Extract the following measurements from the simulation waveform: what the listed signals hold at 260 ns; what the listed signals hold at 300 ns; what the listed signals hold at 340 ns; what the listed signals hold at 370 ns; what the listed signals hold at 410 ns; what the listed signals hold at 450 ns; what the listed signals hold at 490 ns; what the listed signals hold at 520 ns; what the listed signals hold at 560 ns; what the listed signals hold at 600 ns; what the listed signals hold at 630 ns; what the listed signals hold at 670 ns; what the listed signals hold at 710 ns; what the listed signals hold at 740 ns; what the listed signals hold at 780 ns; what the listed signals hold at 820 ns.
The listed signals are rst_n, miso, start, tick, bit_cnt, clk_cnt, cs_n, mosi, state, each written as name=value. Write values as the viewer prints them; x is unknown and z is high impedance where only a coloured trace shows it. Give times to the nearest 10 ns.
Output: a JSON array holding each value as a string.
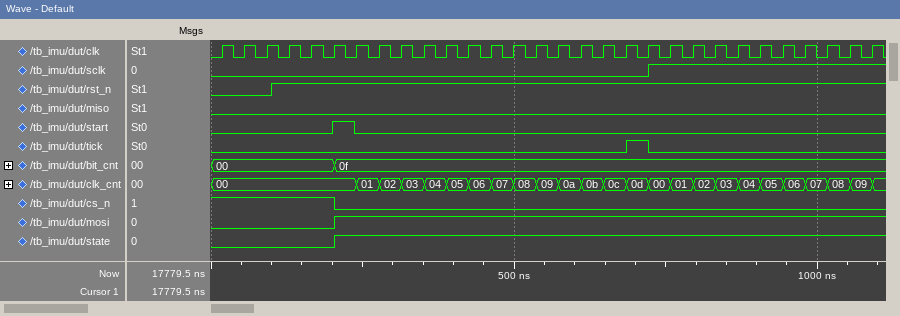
["rst_n=1, miso=0, start=0, tick=0, bit_cnt=0f, clk_cnt=01, cs_n=0, mosi=1, state=1", "rst_n=1, miso=0, start=0, tick=0, bit_cnt=0f, clk_cnt=02, cs_n=0, mosi=1, state=1", "rst_n=1, miso=0, start=0, tick=0, bit_cnt=0f, clk_cnt=03, cs_n=0, mosi=1, state=1", "rst_n=1, miso=0, start=0, tick=0, bit_cnt=0f, clk_cnt=04, cs_n=0, mosi=1, state=1", "rst_n=1, miso=0, start=0, tick=0, bit_cnt=0f, clk_cnt=05, cs_n=0, mosi=1, state=1", "rst_n=1, miso=0, start=0, tick=0, bit_cnt=0f, clk_cnt=06, cs_n=0, mosi=1, state=1", "rst_n=1, miso=0, start=0, tick=0, bit_cnt=0f, clk_cnt=07, cs_n=0, mosi=1, state=1", "rst_n=1, miso=0, start=0, tick=0, bit_cnt=0f, clk_cnt=08, cs_n=0, mosi=1, state=1", "rst_n=1, miso=0, start=0, tick=0, bit_cnt=0f, clk_cnt=09, cs_n=0, mosi=1, state=1", "rst_n=1, miso=0, start=0, tick=0, bit_cnt=0f, clk_cnt=0a, cs_n=0, mosi=1, state=1", "rst_n=1, miso=0, start=0, tick=0, bit_cnt=0f, clk_cnt=0b, cs_n=0, mosi=1, state=1", "rst_n=1, miso=0, start=0, tick=0, bit_cnt=0f, clk_cnt=0c, cs_n=0, mosi=1, state=1", "rst_n=1, miso=0, start=0, tick=1, bit_cnt=0f, clk_cnt=0d, cs_n=0, mosi=1, state=1", "rst_n=1, miso=0, start=0, tick=0, bit_cnt=0f, clk_cnt=00, cs_n=0, mosi=1, state=1", "rst_n=1, miso=0, start=0, tick=0, bit_cnt=0f, clk_cnt=01, cs_n=0, mosi=1, state=1", "rst_n=1, miso=0, start=0, tick=0, bit_cnt=0f, clk_cnt=02, cs_n=0, mosi=1, state=1"]
